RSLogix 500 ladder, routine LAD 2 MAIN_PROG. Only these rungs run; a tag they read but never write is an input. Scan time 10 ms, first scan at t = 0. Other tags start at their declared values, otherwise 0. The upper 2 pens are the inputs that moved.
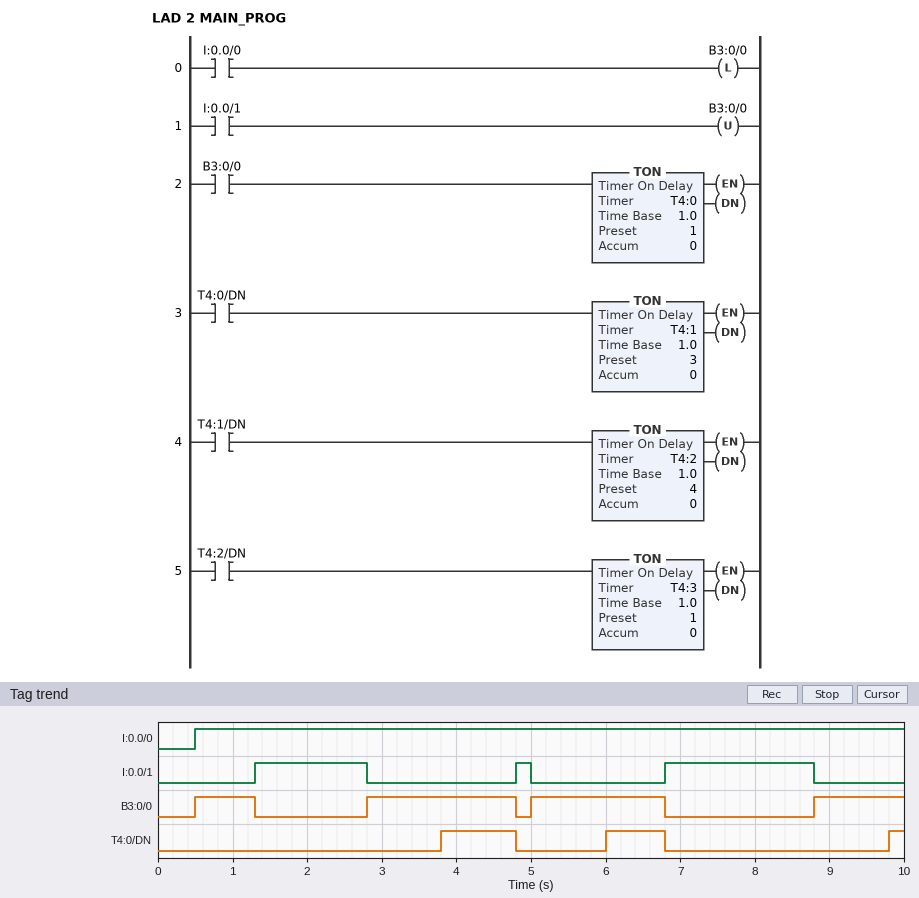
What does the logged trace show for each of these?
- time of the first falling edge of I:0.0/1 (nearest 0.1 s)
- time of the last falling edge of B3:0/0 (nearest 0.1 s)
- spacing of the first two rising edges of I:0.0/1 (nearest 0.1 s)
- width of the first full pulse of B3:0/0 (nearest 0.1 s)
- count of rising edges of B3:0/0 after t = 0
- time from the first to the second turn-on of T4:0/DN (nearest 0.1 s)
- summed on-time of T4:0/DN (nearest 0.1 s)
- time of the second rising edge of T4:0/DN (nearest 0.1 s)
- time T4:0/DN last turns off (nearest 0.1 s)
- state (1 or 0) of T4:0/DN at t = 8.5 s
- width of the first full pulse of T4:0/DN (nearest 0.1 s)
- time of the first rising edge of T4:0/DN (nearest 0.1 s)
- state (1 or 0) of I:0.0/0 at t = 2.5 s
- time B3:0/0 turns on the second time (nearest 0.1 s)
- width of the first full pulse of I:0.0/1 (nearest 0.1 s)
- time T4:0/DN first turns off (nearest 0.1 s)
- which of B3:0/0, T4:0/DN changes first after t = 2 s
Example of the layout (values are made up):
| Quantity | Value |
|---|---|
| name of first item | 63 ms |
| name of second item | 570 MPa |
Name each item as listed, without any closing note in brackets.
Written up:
| Quantity | Value |
|---|---|
| time of the first falling edge of I:0.0/1 | 2.8 s |
| time of the last falling edge of B3:0/0 | 6.8 s |
| spacing of the first two rising edges of I:0.0/1 | 3.5 s |
| width of the first full pulse of B3:0/0 | 0.8 s |
| count of rising edges of B3:0/0 after t = 0 | 4 |
| time from the first to the second turn-on of T4:0/DN | 2.2 s |
| summed on-time of T4:0/DN | 2.0 s |
| time of the second rising edge of T4:0/DN | 6.0 s |
| time T4:0/DN last turns off | 6.8 s |
| state (1 or 0) of T4:0/DN at t = 8.5 s | 0 |
| width of the first full pulse of T4:0/DN | 1.0 s |
| time of the first rising edge of T4:0/DN | 3.8 s |
| state (1 or 0) of I:0.0/0 at t = 2.5 s | 1 |
| time B3:0/0 turns on the second time | 2.8 s |
| width of the first full pulse of I:0.0/1 | 1.5 s |
| time T4:0/DN first turns off | 4.8 s |
| which of B3:0/0, T4:0/DN changes first after t = 2 s | B3:0/0 |
